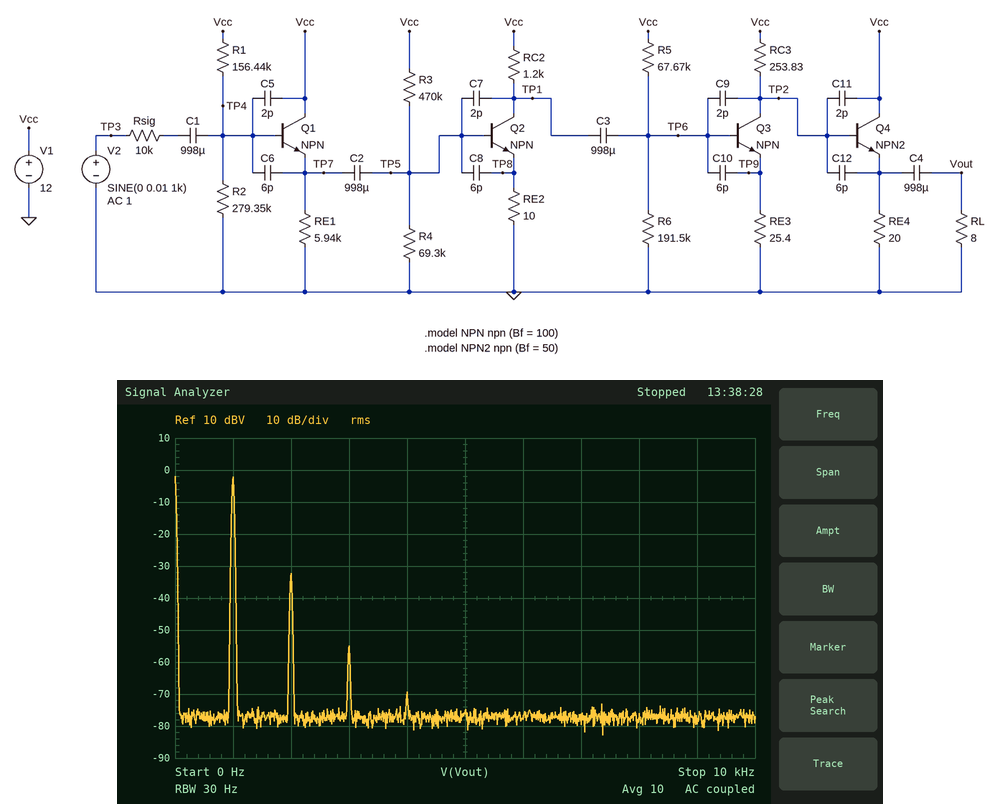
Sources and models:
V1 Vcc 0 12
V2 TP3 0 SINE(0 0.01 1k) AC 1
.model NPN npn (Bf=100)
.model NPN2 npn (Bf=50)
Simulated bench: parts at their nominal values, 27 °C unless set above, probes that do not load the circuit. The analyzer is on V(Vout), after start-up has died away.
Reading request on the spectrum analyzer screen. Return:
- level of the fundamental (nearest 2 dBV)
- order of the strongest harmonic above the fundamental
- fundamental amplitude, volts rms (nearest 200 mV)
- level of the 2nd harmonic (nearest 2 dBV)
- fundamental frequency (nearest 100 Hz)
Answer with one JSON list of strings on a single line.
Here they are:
["-2 dBV", "2", "800 mV", "-32 dBV", "1.0 kHz"]
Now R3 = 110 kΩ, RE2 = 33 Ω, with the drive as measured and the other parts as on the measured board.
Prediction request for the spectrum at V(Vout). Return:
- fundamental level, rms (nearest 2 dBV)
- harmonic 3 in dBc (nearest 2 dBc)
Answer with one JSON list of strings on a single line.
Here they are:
["-4 dBV", "-58 dBc"]
